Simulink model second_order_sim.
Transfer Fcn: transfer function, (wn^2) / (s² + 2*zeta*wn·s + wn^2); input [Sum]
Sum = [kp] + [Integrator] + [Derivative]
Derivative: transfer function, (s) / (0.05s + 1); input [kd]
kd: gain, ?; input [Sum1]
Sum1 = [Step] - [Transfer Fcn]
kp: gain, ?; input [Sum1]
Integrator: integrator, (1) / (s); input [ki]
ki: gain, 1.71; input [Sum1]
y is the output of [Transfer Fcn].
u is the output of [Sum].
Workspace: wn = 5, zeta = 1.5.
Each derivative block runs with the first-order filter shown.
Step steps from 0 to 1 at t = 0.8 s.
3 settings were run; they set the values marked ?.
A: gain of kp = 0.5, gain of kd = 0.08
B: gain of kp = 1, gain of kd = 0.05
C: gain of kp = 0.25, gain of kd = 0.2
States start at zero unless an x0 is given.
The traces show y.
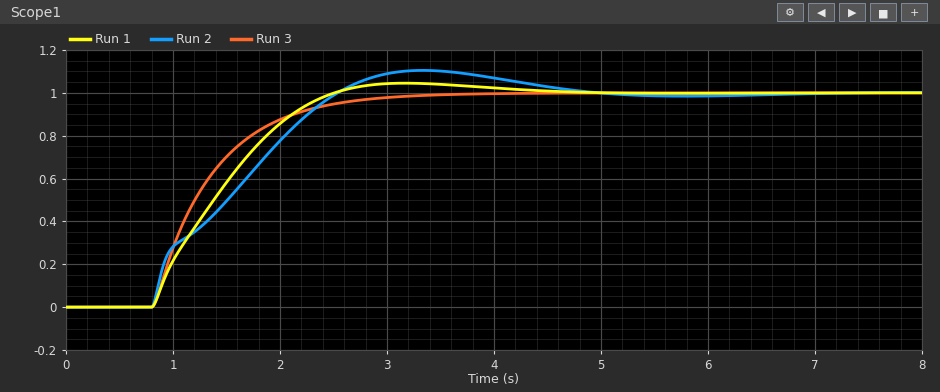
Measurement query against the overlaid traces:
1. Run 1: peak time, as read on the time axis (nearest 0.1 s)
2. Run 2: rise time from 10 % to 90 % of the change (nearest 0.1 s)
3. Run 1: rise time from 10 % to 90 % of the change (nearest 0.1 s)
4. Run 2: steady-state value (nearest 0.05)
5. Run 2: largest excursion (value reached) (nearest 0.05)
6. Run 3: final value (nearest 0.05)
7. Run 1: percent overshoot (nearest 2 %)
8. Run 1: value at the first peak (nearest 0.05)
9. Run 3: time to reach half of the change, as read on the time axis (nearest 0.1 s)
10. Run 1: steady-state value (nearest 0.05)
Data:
3.2 s
1.4 s
1.2 s
1.00
1.10
1.00
4 %
1.05
1.2 s
1.00
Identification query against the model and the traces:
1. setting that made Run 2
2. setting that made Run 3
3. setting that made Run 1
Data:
C
B
A
